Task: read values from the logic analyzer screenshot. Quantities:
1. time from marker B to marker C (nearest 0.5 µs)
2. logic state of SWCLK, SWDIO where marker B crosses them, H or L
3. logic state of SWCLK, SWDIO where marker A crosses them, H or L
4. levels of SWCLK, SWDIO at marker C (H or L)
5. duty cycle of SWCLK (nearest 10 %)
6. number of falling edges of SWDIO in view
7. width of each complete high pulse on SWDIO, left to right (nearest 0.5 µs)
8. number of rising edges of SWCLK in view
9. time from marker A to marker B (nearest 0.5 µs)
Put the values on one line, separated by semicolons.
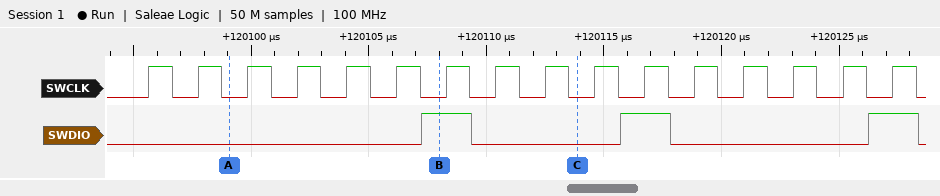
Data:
6 µs; SWCLK=L, SWDIO=H; SWCLK=L, SWDIO=L; SWCLK=L, SWDIO=L; 50 %; 3; 2 µs, 2 µs, 2 µs; 16; 9 µs
